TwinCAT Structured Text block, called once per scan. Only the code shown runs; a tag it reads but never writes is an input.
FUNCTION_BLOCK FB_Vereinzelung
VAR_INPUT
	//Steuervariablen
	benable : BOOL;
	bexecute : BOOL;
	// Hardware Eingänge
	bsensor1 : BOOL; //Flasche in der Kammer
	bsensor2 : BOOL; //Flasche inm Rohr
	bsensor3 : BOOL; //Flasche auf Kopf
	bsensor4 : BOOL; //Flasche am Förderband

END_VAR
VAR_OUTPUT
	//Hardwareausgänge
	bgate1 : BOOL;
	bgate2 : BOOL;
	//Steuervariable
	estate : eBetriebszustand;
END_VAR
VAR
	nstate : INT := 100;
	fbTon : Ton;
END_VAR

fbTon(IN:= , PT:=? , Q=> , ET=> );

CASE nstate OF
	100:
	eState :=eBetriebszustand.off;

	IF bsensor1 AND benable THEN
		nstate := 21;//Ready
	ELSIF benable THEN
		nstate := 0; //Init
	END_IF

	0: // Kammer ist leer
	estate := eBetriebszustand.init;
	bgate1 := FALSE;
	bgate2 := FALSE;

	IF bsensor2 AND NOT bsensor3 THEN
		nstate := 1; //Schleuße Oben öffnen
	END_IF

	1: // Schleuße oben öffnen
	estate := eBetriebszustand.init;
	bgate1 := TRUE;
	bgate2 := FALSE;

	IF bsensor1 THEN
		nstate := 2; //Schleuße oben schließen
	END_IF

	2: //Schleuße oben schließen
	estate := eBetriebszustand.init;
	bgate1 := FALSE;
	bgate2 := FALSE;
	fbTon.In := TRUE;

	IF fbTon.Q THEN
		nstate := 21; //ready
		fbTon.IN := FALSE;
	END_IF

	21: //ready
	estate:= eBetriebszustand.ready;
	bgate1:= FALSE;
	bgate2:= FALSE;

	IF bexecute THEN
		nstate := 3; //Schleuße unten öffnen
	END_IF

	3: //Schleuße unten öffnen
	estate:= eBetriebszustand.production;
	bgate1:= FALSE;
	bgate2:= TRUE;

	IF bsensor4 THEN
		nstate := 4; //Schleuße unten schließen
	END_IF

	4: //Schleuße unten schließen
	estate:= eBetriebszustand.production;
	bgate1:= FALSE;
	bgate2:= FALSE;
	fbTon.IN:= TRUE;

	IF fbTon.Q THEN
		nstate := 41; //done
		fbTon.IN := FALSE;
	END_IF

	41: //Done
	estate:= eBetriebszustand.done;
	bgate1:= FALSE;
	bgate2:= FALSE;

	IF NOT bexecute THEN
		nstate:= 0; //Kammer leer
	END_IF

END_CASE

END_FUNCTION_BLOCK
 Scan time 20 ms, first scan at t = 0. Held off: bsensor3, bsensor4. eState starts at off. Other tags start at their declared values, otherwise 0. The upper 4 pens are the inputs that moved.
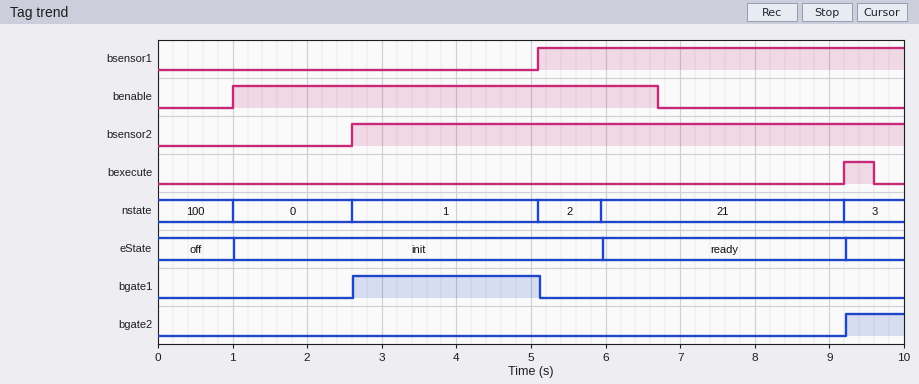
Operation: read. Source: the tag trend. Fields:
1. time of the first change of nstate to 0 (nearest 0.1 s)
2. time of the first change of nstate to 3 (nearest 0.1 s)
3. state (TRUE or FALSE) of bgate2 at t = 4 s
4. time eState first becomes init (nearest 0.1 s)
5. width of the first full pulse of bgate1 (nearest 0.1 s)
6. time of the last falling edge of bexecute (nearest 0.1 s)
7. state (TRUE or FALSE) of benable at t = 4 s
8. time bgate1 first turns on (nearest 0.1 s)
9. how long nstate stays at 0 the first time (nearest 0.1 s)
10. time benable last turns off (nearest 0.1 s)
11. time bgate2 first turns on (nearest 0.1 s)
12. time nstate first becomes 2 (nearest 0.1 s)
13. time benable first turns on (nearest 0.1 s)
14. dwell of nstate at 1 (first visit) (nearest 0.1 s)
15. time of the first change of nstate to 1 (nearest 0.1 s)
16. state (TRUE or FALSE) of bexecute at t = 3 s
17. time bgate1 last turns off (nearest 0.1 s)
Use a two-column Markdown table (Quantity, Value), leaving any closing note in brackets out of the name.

| Quantity | Value |
|---|---|
| time of the first change of nstate to 0 | 1.0 s |
| time of the first change of nstate to 3 | 9.2 s |
| state (TRUE or FALSE) of bgate2 at t = 4 s | FALSE |
| time eState first becomes init | 1.0 s |
| width of the first full pulse of bgate1 | 2.5 s |
| time of the last falling edge of bexecute | 9.6 s |
| state (TRUE or FALSE) of benable at t = 4 s | TRUE |
| time bgate1 first turns on | 2.6 s |
| how long nstate stays at 0 the first time | 1.6 s |
| time benable last turns off | 6.7 s |
| time bgate2 first turns on | 9.2 s |
| time nstate first becomes 2 | 5.1 s |
| time benable first turns on | 1.0 s |
| dwell of nstate at 1 (first visit) | 2.5 s |
| time of the first change of nstate to 1 | 2.6 s |
| state (TRUE or FALSE) of bexecute at t = 3 s | FALSE |
| time bgate1 last turns off | 5.1 s |
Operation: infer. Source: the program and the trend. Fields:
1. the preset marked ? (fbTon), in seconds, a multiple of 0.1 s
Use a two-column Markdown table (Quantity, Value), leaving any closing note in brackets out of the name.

| Quantity | Value |
|---|---|
| the preset marked ? (fbTon), in seconds, a multiple of 0.1 s | 0.8 s |
